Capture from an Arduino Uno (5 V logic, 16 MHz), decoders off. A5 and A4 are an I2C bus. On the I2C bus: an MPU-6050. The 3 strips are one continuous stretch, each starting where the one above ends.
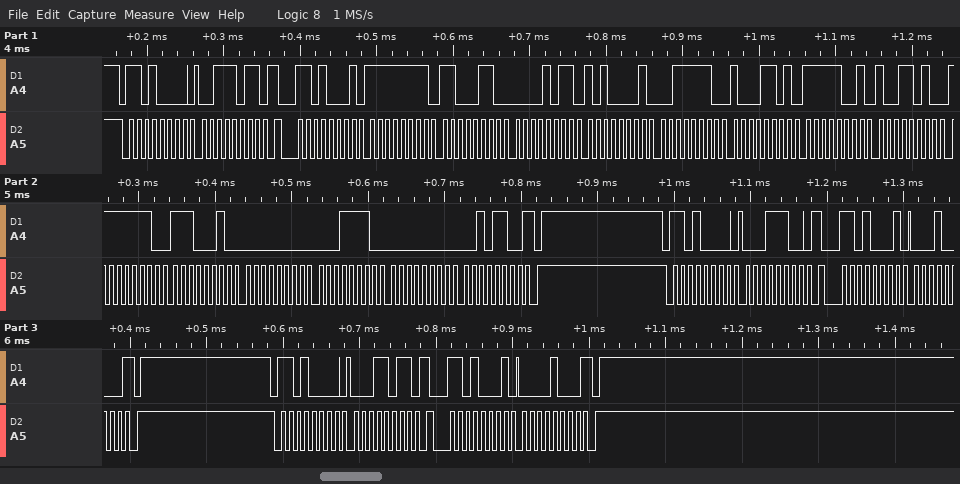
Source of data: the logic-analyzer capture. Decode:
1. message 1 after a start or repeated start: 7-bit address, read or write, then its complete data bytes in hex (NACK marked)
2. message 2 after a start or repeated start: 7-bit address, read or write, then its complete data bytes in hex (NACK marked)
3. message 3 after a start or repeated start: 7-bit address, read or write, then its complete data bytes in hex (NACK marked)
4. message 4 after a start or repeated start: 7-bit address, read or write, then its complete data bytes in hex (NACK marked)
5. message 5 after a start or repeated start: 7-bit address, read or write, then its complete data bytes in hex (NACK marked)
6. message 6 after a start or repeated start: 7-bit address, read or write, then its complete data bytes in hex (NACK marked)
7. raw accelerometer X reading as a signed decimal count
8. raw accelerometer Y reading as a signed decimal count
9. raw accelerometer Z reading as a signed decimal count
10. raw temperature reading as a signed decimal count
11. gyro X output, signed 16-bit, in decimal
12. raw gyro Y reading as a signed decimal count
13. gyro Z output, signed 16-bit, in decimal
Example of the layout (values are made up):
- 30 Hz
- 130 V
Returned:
- 0x68 write: 3B
- 0x68 read: FF C6 0B A1 3E 8D F9 9A FE E2 00 1E 00 2C NACK
- 0x68 write: 1C
- 0x68 read: 10 NACK
- 0x68 write: 1B
- 0x68 read: 08 NACK
- -58
- 2977
- 16013
- -1638
- -286
- 30
- 44
